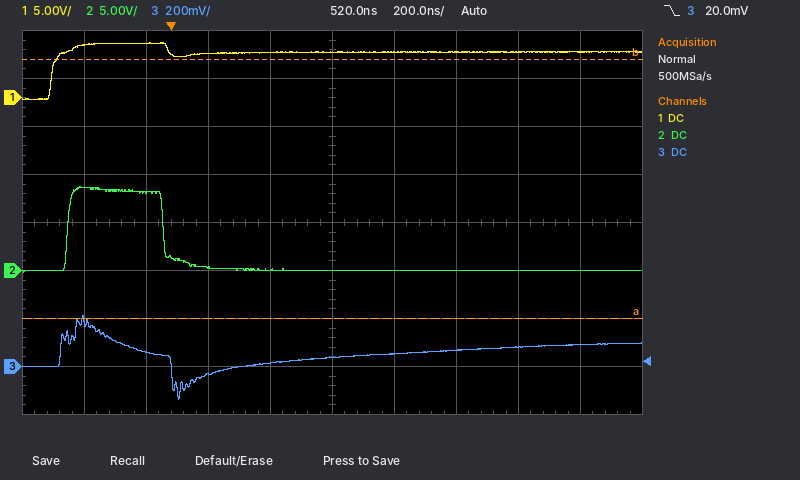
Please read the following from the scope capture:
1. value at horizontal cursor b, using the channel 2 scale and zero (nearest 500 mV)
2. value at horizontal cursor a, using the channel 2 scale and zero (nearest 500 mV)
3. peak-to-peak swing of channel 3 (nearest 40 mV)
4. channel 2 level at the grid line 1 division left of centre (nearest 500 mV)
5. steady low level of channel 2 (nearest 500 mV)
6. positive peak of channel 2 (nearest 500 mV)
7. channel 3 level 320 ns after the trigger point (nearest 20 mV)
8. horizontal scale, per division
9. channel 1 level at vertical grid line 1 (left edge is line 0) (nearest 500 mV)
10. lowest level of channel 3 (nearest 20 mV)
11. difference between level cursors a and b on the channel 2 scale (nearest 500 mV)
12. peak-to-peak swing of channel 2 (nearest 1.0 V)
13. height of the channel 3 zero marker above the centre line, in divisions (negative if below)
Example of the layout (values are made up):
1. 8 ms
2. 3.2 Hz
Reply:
1. 22.0 V
2. -5.0 V
3. 360 mV
4. 0.0 V
5. 0.0 V
6. 9.0 V
7. 20 mV
8. 200 ns
9. 5.5 V
10. -140 mV
11. 27.0 V
12. 9.0 V
13. -3.0 div
